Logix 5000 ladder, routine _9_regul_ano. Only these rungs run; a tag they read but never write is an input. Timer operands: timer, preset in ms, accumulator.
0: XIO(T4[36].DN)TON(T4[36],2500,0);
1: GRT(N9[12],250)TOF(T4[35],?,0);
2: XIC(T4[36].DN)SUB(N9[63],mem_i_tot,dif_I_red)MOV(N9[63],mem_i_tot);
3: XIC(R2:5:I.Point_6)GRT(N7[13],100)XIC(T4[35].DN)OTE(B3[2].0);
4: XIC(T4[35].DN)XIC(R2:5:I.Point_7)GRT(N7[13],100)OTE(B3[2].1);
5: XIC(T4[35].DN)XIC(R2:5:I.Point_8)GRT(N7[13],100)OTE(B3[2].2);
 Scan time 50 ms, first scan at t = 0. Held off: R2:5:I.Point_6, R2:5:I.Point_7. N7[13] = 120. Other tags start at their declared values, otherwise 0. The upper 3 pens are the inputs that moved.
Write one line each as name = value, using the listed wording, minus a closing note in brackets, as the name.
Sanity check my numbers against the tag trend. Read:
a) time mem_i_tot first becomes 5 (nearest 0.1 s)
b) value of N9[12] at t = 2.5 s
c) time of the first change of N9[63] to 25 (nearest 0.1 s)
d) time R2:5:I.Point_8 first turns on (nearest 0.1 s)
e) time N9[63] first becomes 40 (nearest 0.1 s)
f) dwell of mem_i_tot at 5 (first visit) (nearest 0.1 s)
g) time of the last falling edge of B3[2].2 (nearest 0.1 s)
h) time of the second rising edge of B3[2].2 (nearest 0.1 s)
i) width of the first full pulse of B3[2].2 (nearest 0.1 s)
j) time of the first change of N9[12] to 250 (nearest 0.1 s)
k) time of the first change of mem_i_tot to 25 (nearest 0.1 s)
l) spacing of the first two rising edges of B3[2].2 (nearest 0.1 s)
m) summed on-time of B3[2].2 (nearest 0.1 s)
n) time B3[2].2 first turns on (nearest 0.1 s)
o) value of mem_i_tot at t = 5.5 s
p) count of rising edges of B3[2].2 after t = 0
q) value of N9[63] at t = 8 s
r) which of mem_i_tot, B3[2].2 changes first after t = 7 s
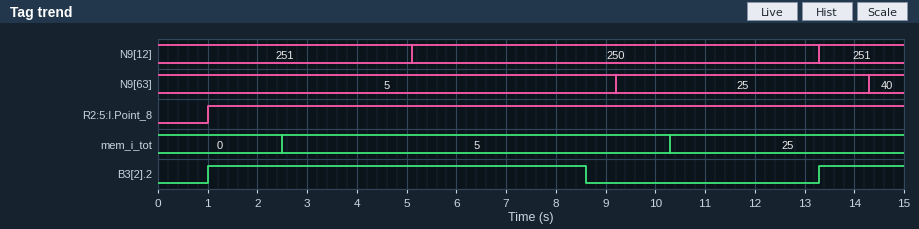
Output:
time mem_i_tot first becomes 5 = 2.5 s
value of N9[12] at t = 2.5 s = 251
time of the first change of N9[63] to 25 = 9.2 s
time R2:5:I.Point_8 first turns on = 1.0 s
time N9[63] first becomes 40 = 14.3 s
dwell of mem_i_tot at 5 (first visit) = 7.8 s
time of the last falling edge of B3[2].2 = 8.6 s
time of the second rising edge of B3[2].2 = 13.3 s
width of the first full pulse of B3[2].2 = 7.6 s
time of the first change of N9[12] to 250 = 5.1 s
time of the first change of mem_i_tot to 25 = 10.3 s
spacing of the first two rising edges of B3[2].2 = 12.3 s
summed on-time of B3[2].2 = 9.3 s
time B3[2].2 first turns on = 1.0 s
value of mem_i_tot at t = 5.5 s = 5
count of rising edges of B3[2].2 after t = 0 = 2
value of N9[63] at t = 8 s = 5
which of mem_i_tot, B3[2].2 changes first after t = 7 s = B3[2].2
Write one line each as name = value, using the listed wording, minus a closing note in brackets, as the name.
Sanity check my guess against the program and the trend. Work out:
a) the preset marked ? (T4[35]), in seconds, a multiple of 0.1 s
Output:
the preset marked ? (T4[35]), in seconds, a multiple of 0.1 s = 3.5 s
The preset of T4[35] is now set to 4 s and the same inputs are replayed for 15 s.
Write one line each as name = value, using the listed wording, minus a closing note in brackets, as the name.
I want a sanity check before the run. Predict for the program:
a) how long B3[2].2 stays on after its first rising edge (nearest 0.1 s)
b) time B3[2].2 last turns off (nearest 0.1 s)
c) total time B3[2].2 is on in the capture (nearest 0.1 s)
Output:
how long B3[2].2 stays on after its first rising edge = 8.1 s
time B3[2].2 last turns off = 9.1 s
total time B3[2].2 is on in the capture = 9.8 s
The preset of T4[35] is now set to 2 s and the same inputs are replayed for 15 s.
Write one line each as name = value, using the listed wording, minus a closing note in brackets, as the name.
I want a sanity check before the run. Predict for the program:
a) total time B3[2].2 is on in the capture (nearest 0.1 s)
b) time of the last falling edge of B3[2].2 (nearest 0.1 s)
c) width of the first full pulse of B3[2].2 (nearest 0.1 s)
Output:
total time B3[2].2 is on in the capture = 7.8 s
time of the last falling edge of B3[2].2 = 7.1 s
width of the first full pulse of B3[2].2 = 6.1 s
